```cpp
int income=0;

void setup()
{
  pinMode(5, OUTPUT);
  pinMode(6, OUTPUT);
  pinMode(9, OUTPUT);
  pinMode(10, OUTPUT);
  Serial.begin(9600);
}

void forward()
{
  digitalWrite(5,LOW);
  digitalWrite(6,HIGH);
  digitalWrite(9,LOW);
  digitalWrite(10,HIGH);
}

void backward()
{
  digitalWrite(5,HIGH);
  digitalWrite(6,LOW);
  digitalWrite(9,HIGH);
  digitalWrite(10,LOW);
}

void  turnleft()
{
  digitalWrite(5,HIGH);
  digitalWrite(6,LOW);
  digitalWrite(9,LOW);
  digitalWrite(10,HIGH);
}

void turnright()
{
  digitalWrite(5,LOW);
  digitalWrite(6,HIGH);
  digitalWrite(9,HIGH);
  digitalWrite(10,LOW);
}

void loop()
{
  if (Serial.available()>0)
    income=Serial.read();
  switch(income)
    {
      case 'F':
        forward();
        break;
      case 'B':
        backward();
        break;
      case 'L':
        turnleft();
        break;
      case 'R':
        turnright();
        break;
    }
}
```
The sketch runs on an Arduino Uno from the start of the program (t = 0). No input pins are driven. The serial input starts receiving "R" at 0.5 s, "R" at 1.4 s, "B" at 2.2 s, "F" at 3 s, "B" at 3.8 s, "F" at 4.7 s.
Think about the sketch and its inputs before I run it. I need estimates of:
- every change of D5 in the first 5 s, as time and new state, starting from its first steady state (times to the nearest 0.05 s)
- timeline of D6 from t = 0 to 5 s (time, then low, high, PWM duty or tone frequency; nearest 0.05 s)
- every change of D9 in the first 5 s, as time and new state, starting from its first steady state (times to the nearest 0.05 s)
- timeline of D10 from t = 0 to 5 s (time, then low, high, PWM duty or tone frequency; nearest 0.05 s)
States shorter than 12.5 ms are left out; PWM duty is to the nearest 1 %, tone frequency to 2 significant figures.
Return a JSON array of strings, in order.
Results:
["0 s low; 2.2 s high; 3 s low; 3.8 s high; 4.7 s low", "0 s low; 0.5 s high; 2.2 s low; 3 s high; 3.8 s low; 4.7 s high", "0 s low; 0.5 s high; 3 s low; 3.8 s high; 4.7 s low", "0 s low; 3 s high; 3.8 s low; 4.7 s high"]
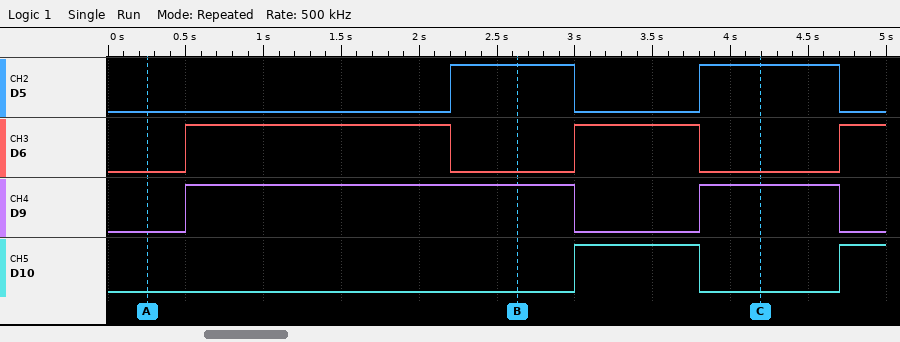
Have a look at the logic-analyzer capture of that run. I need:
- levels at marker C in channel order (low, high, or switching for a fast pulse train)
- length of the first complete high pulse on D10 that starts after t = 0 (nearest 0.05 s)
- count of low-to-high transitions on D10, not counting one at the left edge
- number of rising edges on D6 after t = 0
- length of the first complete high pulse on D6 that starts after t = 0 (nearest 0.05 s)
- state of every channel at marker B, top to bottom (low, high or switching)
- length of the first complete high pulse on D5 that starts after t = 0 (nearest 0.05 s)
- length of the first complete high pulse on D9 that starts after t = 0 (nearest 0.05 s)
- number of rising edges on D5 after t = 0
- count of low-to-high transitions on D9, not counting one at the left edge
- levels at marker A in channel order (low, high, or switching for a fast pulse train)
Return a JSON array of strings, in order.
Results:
["D5 high, D6 low, D9 high, D10 low", "0.80 s", "2", "3", "1.70 s", "D5 high, D6 low, D9 high, D10 low", "0.80 s", "2.50 s", "2", "2", "D5 low, D6 low, D9 low, D10 low"]
